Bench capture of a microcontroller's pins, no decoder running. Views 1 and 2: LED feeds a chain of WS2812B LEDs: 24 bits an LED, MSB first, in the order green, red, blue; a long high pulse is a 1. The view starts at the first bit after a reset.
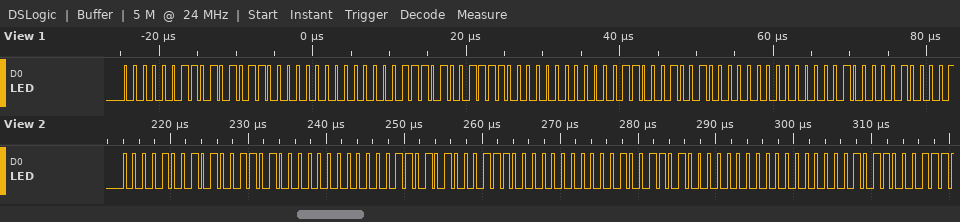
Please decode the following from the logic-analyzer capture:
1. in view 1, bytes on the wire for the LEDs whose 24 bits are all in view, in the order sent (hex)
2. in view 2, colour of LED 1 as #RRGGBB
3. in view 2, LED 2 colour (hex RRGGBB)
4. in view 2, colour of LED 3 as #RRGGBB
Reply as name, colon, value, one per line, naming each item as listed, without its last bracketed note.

in view 1, bytes on the wire for the LEDs whose 24 bits are all in view, in the order sent: 03 56 00 07 4F 00 0C 48 00
in view 2, colour of LED 1 as #RRGGBB: #4D0900
in view 2, LED 2 colour: #470D00
in view 2, colour of LED 3 as #RRGGBB: #401300
